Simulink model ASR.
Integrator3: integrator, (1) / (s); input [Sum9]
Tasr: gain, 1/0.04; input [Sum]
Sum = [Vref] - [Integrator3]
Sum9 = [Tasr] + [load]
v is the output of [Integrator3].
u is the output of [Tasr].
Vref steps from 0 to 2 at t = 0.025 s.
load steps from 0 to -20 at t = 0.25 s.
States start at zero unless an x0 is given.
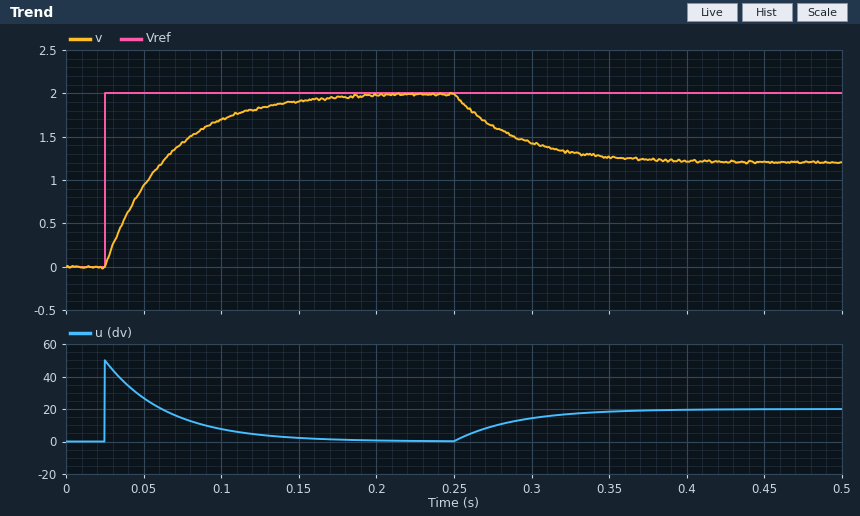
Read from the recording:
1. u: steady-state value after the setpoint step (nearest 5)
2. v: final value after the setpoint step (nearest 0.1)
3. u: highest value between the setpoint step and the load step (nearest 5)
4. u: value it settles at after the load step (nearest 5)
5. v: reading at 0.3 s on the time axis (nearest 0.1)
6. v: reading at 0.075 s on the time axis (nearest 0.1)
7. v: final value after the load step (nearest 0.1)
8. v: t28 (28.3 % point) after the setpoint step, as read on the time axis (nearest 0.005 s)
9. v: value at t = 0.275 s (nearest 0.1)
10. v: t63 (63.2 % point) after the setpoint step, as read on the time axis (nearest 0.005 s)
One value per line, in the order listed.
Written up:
0
2.0
50
20
1.4
1.4
1.2
0.040 s
1.6
0.065 s
